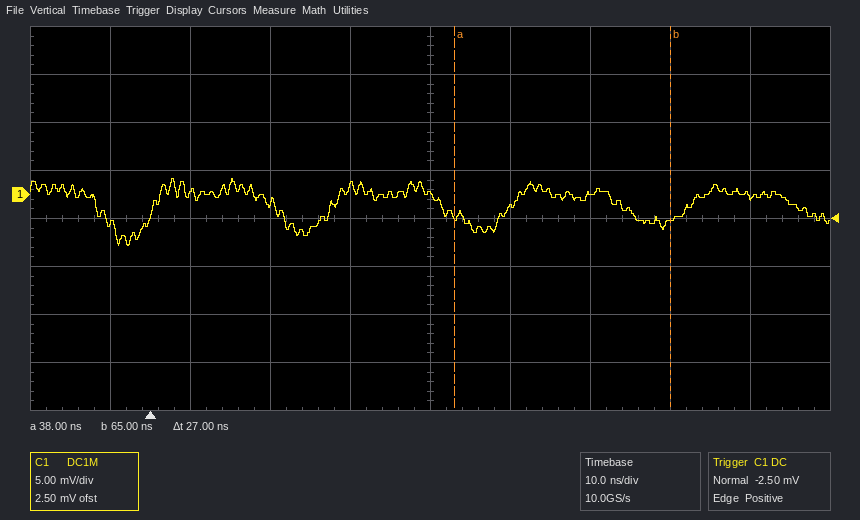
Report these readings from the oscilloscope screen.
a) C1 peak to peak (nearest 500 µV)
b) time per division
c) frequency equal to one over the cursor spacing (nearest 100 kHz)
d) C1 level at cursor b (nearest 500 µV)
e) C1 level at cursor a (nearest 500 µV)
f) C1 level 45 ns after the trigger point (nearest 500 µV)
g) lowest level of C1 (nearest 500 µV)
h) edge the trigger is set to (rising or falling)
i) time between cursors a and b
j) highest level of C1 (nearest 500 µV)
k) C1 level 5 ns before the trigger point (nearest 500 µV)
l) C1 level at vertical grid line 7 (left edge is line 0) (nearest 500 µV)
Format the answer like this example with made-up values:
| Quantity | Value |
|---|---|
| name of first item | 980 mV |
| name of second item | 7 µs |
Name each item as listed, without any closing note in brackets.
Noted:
| Quantity | Value |
|---|---|
| C1 peak to peak | 7.0 mV |
| time per division | 10 ns |
| frequency equal to one over the cursor spacing | 37.0 MHz |
| C1 level at cursor b | -2.5 mV |
| C1 level at cursor a | -2.0 mV |
| C1 level 45 ns after the trigger point | -1.5 mV |
| lowest level of C1 | -5.5 mV |
| edge the trigger is set to | rising |
| time between cursors a and b | 27 ns |
| highest level of C1 | 1.5 mV |
| C1 level 5 ns before the trigger point | -3.0 mV |
| C1 level at vertical grid line 7 (left edge is line 0) | 0.0 mV |
